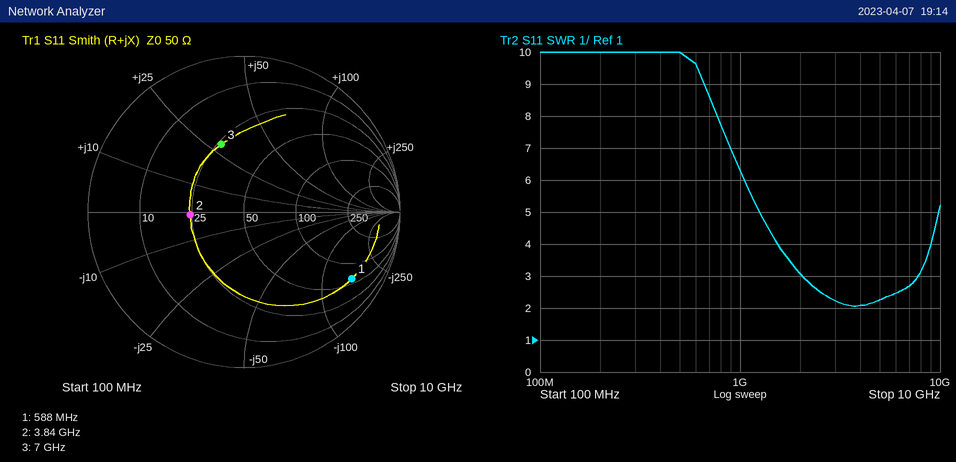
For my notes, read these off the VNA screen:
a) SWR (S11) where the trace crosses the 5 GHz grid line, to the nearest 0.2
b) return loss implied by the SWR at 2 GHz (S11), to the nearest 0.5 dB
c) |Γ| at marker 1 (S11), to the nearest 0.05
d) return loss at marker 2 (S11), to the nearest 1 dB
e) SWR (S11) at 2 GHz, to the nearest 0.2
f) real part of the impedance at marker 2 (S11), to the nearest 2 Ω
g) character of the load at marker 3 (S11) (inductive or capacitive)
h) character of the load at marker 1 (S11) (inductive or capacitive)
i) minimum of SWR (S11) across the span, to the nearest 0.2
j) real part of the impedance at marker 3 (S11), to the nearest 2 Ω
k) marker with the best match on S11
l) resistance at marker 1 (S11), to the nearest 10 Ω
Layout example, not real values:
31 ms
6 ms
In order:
2.2
6.0 dB
0.80
9 dB
3.0
24 Ω
inductive
capacitive
2.0
26 Ω
marker 2
60 Ω
